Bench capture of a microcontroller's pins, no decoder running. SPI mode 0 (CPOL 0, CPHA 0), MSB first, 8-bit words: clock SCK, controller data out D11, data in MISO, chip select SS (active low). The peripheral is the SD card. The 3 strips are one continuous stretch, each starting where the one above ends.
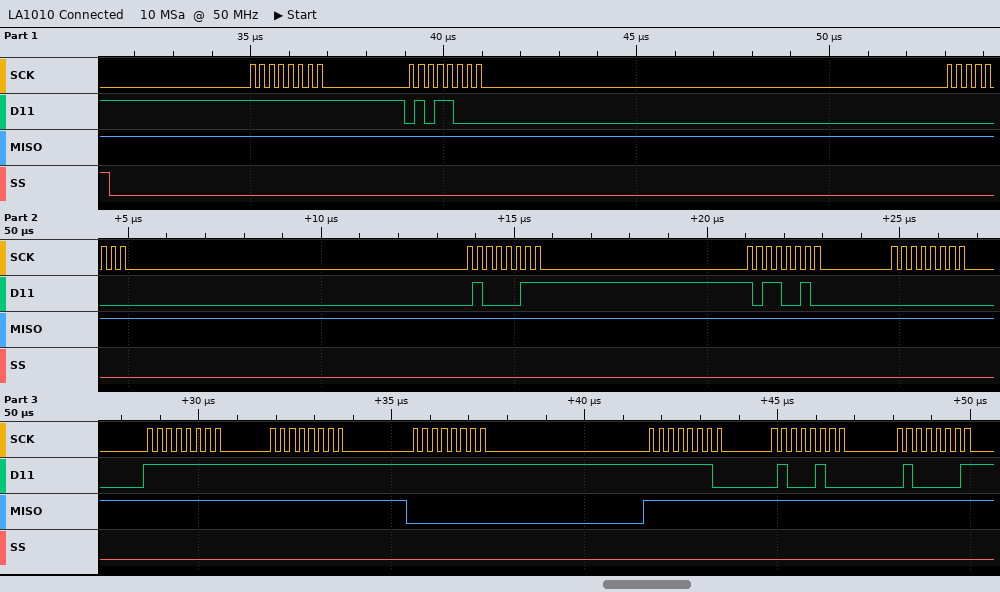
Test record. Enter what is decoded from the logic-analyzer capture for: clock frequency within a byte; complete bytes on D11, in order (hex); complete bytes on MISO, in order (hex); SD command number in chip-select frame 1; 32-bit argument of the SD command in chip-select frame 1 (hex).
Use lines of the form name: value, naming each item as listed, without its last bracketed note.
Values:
clock frequency within a byte: 4 MHz
complete bytes on D11, in order: 0xFF 0x58 0x00 0x43 0xB2 0x00 0xFF 0xFF 0xFF 0xFE 0x44 0x41
complete bytes on MISO, in order: 0xFF 0xFF 0xFF 0xFF 0xFF 0xFF 0xFF 0xFF 0x00 0xFF 0xFF 0xFF
SD command number in chip-select frame 1: CMD24
32-bit argument of the SD command in chip-select frame 1: 0x0043B200
